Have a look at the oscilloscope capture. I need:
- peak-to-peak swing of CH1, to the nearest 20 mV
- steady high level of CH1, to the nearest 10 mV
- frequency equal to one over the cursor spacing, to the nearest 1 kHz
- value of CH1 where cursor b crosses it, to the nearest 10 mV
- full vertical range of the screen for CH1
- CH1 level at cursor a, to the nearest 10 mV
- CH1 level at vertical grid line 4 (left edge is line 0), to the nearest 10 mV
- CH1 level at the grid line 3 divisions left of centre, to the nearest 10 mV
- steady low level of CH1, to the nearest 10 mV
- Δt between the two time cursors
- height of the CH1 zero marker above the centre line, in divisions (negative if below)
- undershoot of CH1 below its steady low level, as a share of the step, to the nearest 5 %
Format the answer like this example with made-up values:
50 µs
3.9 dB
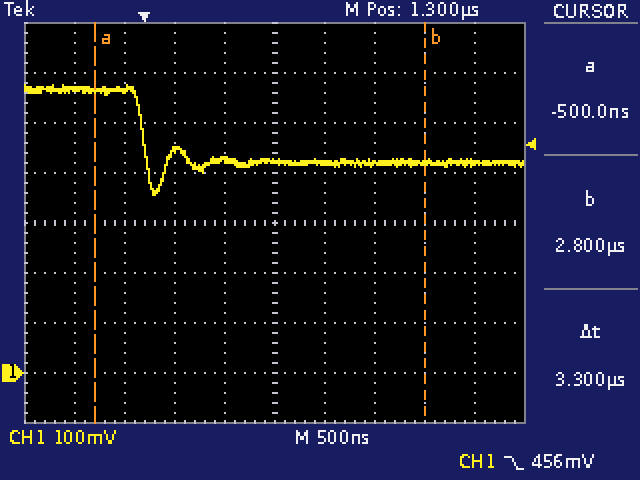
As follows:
220 mV
570 mV
303 kHz
420 mV
800 mV
570 mV
430 mV
570 mV
420 mV
3.3 µs
-3.0 div
45 %
